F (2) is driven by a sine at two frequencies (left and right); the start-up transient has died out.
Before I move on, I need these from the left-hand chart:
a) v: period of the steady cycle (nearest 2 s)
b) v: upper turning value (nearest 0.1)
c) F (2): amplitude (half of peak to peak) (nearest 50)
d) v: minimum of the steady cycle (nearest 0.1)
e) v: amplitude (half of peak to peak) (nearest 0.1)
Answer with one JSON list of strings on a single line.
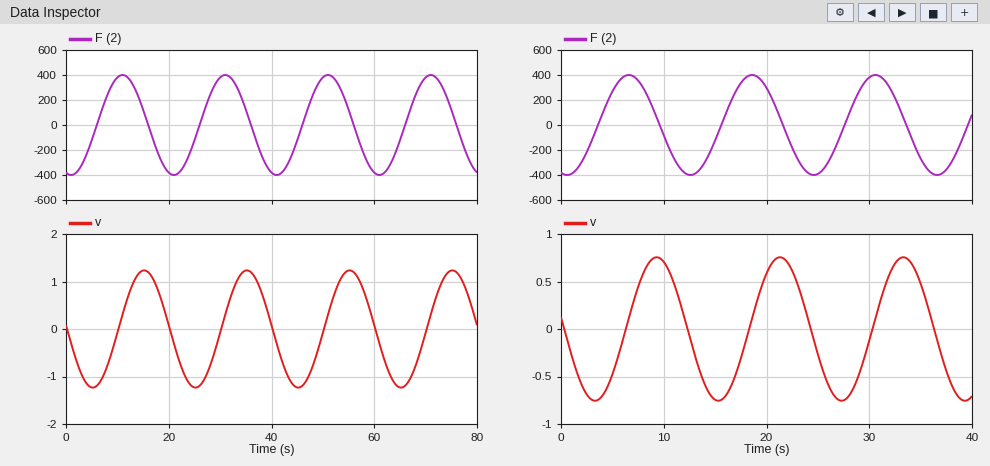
["20 s", "1.2", "400", "-1.2", "1.2"]
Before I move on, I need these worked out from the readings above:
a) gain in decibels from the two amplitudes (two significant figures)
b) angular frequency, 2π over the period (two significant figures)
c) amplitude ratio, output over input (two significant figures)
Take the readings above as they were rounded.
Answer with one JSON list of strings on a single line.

["-50 dB", "0.31 rad/s", "0.0030"]
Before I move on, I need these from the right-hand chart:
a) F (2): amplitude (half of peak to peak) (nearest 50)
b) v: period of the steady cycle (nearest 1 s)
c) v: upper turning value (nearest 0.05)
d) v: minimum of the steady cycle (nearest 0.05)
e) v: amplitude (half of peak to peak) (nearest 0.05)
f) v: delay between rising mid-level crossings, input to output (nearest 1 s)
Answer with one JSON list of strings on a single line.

["400", "12 s", "0.75", "-0.75", "0.75", "3 s"]
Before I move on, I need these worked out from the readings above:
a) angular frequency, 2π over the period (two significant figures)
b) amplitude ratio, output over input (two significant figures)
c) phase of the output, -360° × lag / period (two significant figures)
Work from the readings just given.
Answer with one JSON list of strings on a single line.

["0.52 rad/s", "0.0019", "-90°"]
